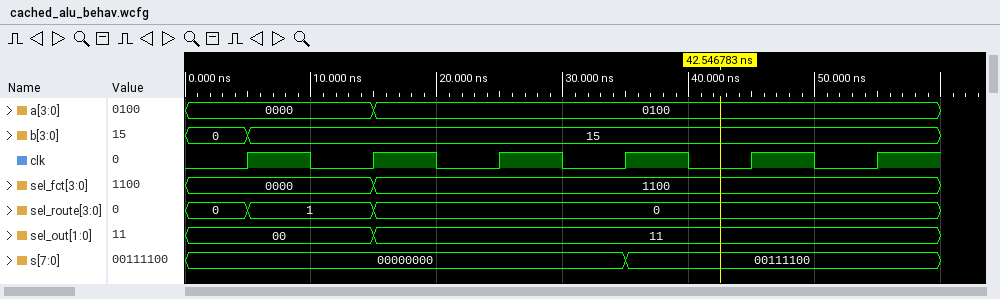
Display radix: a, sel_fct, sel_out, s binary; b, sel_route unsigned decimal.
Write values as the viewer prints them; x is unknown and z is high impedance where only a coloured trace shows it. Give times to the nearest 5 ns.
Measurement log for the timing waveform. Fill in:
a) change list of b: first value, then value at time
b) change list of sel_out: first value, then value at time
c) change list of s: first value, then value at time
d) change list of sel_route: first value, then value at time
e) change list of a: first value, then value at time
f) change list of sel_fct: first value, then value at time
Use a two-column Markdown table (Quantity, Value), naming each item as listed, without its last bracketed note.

| Quantity | Value |
|---|---|
| change list of b: first value, then value at time | 0, 15 at 5 ns |
| change list of sel_out: first value, then value at time | 00, 11 at 15 ns |
| change list of s: first value, then value at time | 00000000, 00111100 at 35 ns |
| change list of sel_route: first value, then value at time | 0, 1 at 5 ns, 0 at 15 ns |
| change list of a: first value, then value at time | 0000, 0100 at 15 ns |
| change list of sel_fct: first value, then value at time | 0000, 1100 at 15 ns |
